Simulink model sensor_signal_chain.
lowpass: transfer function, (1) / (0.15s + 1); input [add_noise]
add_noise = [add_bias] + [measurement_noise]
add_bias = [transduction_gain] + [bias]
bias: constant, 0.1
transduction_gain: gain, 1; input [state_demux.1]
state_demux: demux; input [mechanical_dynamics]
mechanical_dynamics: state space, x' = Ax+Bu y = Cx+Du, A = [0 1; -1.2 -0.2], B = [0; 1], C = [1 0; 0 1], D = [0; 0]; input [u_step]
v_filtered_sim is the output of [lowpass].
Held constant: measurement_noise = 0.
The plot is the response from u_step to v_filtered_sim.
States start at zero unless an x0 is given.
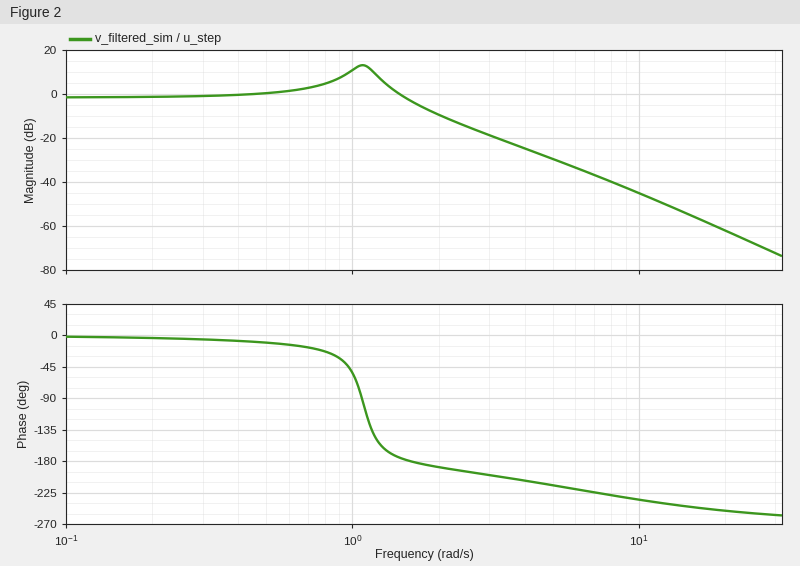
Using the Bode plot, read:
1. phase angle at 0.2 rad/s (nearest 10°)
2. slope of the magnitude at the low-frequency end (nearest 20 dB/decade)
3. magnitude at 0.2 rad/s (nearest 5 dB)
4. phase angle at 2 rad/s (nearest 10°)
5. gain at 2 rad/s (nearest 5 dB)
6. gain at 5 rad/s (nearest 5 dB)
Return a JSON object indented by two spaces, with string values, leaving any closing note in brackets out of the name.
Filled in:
{
  "phase angle at 0.2 rad/s": "0°",
  "slope of the magnitude at the low-frequency end": "0 dB/decade",
  "magnitude at 0.2 rad/s": "0 dB",
  "phase angle at 2 rad/s": "-190°",
  "gain at 2 rad/s": "-10 dB",
  "gain at 5 rad/s": "-30 dB"
}
